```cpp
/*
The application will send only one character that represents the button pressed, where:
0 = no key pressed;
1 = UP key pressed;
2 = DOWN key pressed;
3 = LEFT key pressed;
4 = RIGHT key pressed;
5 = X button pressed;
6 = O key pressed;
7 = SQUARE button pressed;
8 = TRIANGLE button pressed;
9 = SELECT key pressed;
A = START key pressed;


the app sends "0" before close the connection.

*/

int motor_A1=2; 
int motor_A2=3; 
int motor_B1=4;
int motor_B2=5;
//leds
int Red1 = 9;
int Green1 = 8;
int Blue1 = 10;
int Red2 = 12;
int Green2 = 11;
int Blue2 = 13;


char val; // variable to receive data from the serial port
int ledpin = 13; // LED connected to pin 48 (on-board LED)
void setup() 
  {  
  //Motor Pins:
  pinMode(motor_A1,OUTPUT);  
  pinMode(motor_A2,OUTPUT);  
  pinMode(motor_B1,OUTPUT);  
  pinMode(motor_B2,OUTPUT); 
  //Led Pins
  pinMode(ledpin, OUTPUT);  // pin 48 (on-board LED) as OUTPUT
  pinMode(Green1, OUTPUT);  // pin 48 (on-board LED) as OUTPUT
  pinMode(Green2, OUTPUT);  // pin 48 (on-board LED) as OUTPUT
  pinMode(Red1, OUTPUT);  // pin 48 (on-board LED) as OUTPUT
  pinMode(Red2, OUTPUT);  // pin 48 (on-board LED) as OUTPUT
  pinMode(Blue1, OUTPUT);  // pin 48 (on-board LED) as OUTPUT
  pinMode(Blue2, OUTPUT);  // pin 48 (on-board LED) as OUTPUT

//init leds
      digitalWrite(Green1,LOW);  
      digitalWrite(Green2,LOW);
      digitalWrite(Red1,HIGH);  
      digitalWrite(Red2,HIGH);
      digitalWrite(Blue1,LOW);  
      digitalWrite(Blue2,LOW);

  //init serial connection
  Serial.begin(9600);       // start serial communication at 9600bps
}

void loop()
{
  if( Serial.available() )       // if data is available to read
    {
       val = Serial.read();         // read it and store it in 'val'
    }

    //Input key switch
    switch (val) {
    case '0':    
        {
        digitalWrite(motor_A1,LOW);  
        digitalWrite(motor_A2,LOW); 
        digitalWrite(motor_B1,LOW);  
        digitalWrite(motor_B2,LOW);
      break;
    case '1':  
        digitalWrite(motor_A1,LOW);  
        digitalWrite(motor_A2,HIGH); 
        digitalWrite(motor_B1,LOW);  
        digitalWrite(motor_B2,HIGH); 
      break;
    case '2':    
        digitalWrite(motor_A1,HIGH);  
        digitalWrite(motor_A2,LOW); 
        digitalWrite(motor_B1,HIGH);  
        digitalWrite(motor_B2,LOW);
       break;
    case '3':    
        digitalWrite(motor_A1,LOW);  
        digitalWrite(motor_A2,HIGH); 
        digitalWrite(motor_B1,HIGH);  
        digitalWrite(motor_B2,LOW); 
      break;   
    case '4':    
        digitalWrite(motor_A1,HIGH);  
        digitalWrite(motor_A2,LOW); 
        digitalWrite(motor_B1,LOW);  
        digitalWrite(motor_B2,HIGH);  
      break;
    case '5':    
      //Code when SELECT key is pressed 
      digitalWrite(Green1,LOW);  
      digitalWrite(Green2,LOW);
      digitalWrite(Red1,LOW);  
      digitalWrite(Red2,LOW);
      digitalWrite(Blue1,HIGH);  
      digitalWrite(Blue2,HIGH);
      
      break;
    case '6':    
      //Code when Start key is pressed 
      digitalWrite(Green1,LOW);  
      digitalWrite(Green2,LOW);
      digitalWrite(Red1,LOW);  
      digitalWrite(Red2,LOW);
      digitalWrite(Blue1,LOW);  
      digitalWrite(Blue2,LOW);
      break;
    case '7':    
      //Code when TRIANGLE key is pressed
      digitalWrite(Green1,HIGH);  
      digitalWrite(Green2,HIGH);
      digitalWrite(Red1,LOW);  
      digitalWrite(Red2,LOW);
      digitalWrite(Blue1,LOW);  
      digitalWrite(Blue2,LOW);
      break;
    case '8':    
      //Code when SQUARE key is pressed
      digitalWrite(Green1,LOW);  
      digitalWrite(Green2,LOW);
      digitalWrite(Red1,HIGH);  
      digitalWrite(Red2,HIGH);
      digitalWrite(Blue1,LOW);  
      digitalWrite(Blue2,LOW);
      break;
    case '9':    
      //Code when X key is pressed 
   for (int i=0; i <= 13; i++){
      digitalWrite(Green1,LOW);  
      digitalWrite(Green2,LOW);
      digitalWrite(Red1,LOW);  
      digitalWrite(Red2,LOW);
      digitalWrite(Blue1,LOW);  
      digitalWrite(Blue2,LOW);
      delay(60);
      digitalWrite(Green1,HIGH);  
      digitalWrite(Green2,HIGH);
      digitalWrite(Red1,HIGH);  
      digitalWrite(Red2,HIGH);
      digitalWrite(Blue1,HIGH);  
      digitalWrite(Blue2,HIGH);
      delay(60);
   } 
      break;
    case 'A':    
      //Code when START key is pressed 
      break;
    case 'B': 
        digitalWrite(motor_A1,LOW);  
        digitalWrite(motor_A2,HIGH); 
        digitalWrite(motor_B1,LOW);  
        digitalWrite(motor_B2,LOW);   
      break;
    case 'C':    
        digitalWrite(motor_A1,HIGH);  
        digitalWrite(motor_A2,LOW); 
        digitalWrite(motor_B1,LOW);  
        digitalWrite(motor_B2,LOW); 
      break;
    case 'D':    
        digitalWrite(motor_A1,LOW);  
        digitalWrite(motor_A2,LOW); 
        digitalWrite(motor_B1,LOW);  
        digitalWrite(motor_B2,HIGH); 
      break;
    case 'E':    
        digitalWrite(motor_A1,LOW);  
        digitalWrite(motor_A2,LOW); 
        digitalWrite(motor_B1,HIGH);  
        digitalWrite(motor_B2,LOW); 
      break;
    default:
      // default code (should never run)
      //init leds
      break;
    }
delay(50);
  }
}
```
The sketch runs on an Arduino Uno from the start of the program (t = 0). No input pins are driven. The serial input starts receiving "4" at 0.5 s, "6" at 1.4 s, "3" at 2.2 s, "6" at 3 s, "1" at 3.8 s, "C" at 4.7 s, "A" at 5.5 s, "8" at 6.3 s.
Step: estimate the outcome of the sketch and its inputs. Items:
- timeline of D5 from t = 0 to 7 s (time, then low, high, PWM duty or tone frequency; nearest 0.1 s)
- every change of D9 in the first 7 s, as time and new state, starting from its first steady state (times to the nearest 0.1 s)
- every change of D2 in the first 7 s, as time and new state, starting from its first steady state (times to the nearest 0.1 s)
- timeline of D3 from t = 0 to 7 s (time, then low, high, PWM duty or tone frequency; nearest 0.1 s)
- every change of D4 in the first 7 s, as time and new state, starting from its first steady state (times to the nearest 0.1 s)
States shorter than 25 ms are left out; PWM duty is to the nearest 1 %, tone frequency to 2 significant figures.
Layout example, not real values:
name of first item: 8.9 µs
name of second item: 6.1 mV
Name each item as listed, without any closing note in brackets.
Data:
timeline of D5 from t = 0 to 7 s: 0 s low; 0.5 s high; 2.2 s low; 3.8 s high; 4.7 s low
every change of D9 in the first 7 s, as time and new state, starting from its first steady state: 0 s high; 1.4 s low; 6.3 s high
every change of D2 in the first 7 s, as time and new state, starting from its first steady state: 0 s low; 0.5 s high; 2.2 s low; 4.7 s high
timeline of D3 from t = 0 to 7 s: 0 s low; 2.2 s high; 4.7 s low
every change of D4 in the first 7 s, as time and new state, starting from its first steady state: 0 s low; 2.2 s high; 3.8 s low
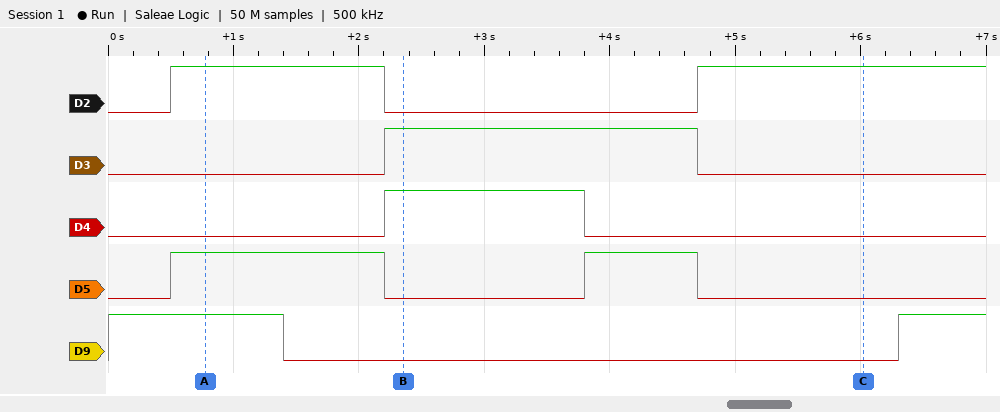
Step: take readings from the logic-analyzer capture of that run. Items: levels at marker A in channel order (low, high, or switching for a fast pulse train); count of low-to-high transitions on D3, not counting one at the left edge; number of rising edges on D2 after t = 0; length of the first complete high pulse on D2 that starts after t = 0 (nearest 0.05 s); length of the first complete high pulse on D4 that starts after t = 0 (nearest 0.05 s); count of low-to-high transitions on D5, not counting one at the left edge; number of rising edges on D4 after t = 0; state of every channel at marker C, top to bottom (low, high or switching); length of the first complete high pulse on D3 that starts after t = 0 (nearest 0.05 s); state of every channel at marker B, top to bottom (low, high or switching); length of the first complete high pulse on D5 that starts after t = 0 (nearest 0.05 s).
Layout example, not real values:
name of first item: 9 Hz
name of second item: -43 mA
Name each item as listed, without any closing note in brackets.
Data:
levels at marker A in channel order: D2 high, D3 low, D4 low, D5 high, D9 high
count of low-to-high transitions on D3, not counting one at the left edge: 1
number of rising edges on D2 after t = 0: 2
length of the first complete high pulse on D2 that starts after t = 0: 1.70 s
length of the first complete high pulse on D4 that starts after t = 0: 1.60 s
count of low-to-high transitions on D5, not counting one at the left edge: 2
number of rising edges on D4 after t = 0: 1
state of every channel at marker C, top to bottom: D2 high, D3 low, D4 low, D5 low, D9 low
length of the first complete high pulse on D3 that starts after t = 0: 2.50 s
state of every channel at marker B, top to bottom: D2 low, D3 high, D4 high, D5 low, D9 low
length of the first complete high pulse on D5 that starts after t = 0: 1.70 s
